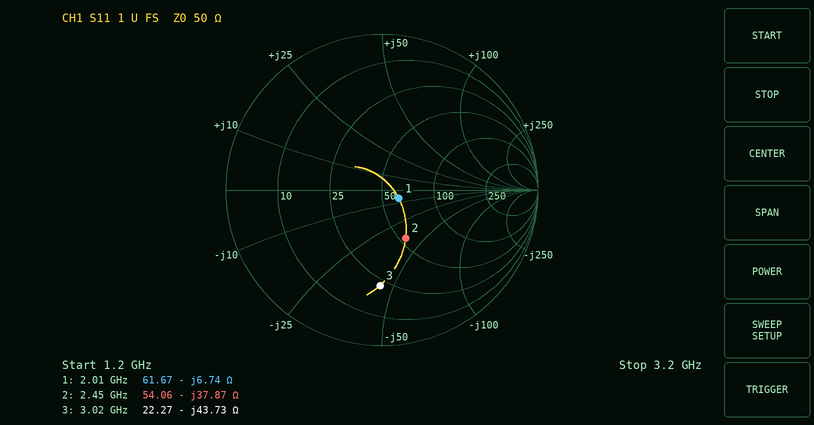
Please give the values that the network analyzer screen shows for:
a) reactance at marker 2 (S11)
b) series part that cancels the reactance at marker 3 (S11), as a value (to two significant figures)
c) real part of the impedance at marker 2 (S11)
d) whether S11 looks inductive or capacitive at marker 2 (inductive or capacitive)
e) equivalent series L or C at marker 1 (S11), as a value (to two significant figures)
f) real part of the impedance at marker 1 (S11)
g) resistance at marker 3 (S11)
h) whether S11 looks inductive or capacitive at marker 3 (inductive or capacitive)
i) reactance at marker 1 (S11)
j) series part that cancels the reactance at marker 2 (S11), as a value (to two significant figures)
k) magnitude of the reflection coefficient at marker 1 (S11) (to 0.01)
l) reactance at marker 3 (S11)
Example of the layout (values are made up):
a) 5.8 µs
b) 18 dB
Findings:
a) -37.87 Ω
b) 2.3 nH
c) 54.06 Ω
d) capacitive
e) 12 pF
f) 61.67 Ω
g) 22.27 Ω
h) capacitive
i) -6.74 Ω
j) 2.5 nH
k) 0.12
l) -43.73 Ω
